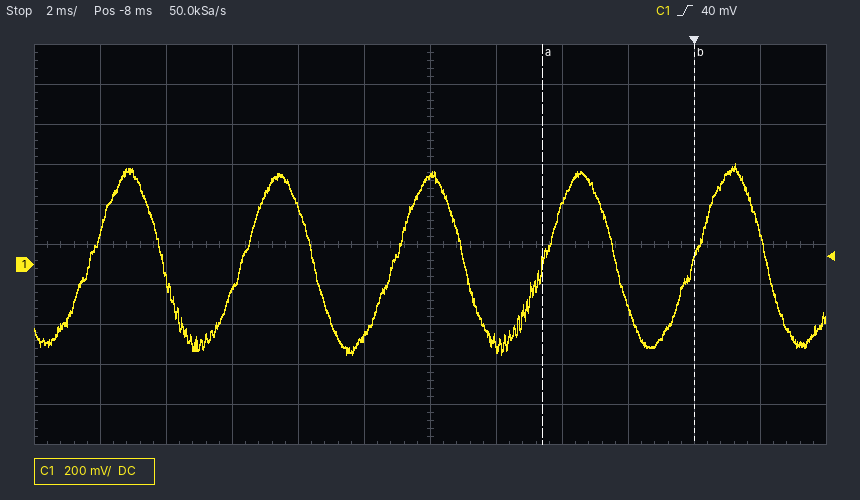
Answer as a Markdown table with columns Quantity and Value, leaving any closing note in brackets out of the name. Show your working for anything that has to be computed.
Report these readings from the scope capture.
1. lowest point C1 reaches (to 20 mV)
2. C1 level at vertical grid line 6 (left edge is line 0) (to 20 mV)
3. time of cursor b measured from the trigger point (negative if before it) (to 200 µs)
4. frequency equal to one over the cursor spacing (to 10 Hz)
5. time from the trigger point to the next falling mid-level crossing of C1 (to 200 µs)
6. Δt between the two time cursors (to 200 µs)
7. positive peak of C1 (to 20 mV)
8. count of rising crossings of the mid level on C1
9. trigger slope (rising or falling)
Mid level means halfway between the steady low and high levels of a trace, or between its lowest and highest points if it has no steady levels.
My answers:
| Quantity | Value |
|---|---|
| lowest point C1 reaches | -440 mV |
| C1 level at vertical grid line 6 (left edge is line 0) | 440 mV |
| time of cursor b measured from the trigger point (negative if before it) | 0.0 ms |
| frequency equal to one over the cursor spacing | 1 / 4.6 ms ≈ 220 Hz |
| time from the trigger point to the next falling mid-level crossing of C1 | 2.2 ms |
| Δt between the two time cursors | 4.6 ms |
| positive peak of C1 | 500 mV |
| count of rising crossings of the mid level on C1 | 5 |
| trigger slope | rising |
